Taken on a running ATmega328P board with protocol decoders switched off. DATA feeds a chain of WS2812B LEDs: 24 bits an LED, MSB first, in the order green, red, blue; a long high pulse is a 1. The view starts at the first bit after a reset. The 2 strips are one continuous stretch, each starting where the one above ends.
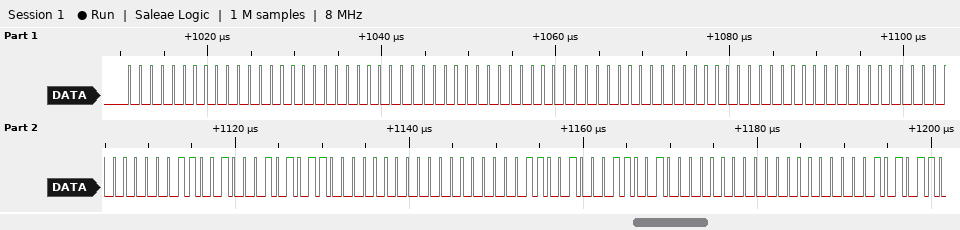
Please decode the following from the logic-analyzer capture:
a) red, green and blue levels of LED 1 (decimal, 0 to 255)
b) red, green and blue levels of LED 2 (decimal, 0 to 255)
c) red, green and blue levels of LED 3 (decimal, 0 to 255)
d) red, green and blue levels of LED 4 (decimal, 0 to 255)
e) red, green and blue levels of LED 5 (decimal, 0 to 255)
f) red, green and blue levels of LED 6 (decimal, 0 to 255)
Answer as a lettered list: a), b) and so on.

a) 0, 0, 0
b) 0, 0, 0
c) 0, 0, 0
d) 50, 0, 43
e) 0, 0, 50
f) 0, 50, 0
